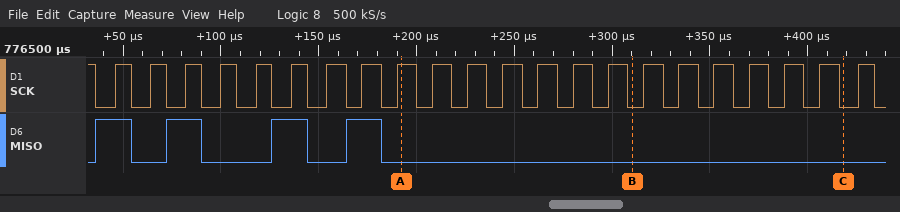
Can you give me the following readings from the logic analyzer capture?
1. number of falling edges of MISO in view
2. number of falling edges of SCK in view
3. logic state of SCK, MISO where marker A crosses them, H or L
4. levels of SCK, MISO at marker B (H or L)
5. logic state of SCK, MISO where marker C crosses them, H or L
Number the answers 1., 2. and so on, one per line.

1. 4
2. 23
3. SCK=H, MISO=L
4. SCK=L, MISO=L
5. SCK=L, MISO=L
